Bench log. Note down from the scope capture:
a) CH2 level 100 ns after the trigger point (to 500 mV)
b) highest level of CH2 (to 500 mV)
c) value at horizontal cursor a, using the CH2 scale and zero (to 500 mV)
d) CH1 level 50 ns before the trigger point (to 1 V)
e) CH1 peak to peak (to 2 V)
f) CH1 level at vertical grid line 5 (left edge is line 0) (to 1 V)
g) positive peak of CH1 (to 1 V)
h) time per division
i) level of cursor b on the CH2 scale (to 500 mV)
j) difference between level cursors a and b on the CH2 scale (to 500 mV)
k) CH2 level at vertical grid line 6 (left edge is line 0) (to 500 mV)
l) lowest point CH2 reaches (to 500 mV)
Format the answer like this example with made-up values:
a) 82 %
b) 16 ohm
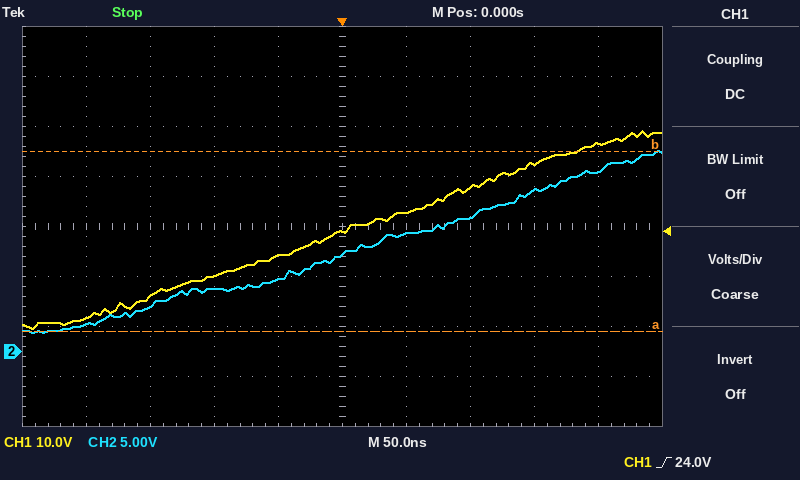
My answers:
a) 13.5 V
b) 20.0 V
c) 2.0 V
d) 19 V
e) 40 V
f) 24 V
g) 44 V
h) 50 ns
i) 20.0 V
j) 18.0 V
k) 12.0 V
l) 2.0 V
